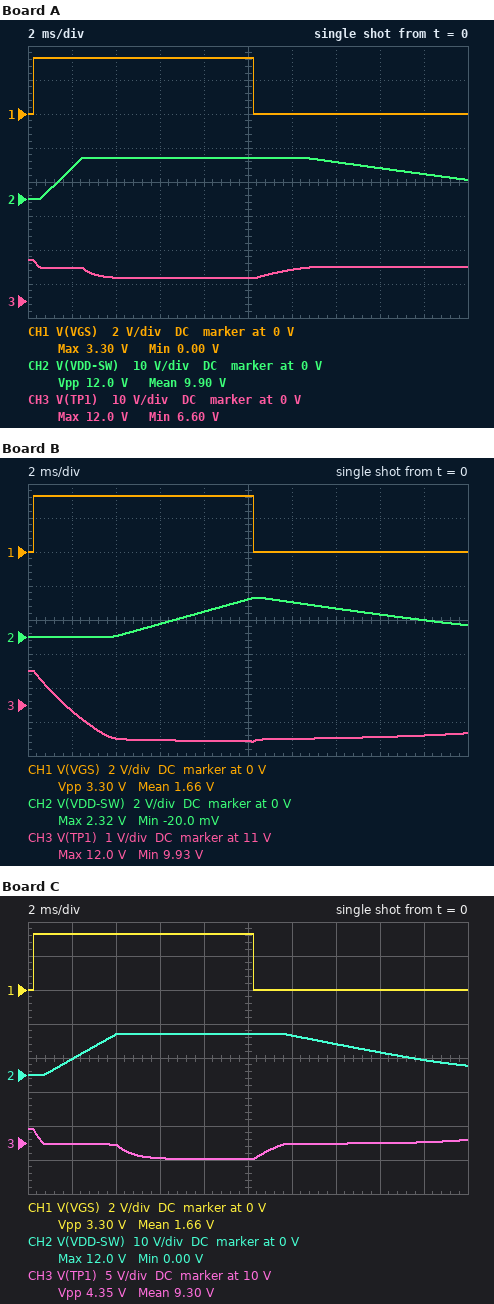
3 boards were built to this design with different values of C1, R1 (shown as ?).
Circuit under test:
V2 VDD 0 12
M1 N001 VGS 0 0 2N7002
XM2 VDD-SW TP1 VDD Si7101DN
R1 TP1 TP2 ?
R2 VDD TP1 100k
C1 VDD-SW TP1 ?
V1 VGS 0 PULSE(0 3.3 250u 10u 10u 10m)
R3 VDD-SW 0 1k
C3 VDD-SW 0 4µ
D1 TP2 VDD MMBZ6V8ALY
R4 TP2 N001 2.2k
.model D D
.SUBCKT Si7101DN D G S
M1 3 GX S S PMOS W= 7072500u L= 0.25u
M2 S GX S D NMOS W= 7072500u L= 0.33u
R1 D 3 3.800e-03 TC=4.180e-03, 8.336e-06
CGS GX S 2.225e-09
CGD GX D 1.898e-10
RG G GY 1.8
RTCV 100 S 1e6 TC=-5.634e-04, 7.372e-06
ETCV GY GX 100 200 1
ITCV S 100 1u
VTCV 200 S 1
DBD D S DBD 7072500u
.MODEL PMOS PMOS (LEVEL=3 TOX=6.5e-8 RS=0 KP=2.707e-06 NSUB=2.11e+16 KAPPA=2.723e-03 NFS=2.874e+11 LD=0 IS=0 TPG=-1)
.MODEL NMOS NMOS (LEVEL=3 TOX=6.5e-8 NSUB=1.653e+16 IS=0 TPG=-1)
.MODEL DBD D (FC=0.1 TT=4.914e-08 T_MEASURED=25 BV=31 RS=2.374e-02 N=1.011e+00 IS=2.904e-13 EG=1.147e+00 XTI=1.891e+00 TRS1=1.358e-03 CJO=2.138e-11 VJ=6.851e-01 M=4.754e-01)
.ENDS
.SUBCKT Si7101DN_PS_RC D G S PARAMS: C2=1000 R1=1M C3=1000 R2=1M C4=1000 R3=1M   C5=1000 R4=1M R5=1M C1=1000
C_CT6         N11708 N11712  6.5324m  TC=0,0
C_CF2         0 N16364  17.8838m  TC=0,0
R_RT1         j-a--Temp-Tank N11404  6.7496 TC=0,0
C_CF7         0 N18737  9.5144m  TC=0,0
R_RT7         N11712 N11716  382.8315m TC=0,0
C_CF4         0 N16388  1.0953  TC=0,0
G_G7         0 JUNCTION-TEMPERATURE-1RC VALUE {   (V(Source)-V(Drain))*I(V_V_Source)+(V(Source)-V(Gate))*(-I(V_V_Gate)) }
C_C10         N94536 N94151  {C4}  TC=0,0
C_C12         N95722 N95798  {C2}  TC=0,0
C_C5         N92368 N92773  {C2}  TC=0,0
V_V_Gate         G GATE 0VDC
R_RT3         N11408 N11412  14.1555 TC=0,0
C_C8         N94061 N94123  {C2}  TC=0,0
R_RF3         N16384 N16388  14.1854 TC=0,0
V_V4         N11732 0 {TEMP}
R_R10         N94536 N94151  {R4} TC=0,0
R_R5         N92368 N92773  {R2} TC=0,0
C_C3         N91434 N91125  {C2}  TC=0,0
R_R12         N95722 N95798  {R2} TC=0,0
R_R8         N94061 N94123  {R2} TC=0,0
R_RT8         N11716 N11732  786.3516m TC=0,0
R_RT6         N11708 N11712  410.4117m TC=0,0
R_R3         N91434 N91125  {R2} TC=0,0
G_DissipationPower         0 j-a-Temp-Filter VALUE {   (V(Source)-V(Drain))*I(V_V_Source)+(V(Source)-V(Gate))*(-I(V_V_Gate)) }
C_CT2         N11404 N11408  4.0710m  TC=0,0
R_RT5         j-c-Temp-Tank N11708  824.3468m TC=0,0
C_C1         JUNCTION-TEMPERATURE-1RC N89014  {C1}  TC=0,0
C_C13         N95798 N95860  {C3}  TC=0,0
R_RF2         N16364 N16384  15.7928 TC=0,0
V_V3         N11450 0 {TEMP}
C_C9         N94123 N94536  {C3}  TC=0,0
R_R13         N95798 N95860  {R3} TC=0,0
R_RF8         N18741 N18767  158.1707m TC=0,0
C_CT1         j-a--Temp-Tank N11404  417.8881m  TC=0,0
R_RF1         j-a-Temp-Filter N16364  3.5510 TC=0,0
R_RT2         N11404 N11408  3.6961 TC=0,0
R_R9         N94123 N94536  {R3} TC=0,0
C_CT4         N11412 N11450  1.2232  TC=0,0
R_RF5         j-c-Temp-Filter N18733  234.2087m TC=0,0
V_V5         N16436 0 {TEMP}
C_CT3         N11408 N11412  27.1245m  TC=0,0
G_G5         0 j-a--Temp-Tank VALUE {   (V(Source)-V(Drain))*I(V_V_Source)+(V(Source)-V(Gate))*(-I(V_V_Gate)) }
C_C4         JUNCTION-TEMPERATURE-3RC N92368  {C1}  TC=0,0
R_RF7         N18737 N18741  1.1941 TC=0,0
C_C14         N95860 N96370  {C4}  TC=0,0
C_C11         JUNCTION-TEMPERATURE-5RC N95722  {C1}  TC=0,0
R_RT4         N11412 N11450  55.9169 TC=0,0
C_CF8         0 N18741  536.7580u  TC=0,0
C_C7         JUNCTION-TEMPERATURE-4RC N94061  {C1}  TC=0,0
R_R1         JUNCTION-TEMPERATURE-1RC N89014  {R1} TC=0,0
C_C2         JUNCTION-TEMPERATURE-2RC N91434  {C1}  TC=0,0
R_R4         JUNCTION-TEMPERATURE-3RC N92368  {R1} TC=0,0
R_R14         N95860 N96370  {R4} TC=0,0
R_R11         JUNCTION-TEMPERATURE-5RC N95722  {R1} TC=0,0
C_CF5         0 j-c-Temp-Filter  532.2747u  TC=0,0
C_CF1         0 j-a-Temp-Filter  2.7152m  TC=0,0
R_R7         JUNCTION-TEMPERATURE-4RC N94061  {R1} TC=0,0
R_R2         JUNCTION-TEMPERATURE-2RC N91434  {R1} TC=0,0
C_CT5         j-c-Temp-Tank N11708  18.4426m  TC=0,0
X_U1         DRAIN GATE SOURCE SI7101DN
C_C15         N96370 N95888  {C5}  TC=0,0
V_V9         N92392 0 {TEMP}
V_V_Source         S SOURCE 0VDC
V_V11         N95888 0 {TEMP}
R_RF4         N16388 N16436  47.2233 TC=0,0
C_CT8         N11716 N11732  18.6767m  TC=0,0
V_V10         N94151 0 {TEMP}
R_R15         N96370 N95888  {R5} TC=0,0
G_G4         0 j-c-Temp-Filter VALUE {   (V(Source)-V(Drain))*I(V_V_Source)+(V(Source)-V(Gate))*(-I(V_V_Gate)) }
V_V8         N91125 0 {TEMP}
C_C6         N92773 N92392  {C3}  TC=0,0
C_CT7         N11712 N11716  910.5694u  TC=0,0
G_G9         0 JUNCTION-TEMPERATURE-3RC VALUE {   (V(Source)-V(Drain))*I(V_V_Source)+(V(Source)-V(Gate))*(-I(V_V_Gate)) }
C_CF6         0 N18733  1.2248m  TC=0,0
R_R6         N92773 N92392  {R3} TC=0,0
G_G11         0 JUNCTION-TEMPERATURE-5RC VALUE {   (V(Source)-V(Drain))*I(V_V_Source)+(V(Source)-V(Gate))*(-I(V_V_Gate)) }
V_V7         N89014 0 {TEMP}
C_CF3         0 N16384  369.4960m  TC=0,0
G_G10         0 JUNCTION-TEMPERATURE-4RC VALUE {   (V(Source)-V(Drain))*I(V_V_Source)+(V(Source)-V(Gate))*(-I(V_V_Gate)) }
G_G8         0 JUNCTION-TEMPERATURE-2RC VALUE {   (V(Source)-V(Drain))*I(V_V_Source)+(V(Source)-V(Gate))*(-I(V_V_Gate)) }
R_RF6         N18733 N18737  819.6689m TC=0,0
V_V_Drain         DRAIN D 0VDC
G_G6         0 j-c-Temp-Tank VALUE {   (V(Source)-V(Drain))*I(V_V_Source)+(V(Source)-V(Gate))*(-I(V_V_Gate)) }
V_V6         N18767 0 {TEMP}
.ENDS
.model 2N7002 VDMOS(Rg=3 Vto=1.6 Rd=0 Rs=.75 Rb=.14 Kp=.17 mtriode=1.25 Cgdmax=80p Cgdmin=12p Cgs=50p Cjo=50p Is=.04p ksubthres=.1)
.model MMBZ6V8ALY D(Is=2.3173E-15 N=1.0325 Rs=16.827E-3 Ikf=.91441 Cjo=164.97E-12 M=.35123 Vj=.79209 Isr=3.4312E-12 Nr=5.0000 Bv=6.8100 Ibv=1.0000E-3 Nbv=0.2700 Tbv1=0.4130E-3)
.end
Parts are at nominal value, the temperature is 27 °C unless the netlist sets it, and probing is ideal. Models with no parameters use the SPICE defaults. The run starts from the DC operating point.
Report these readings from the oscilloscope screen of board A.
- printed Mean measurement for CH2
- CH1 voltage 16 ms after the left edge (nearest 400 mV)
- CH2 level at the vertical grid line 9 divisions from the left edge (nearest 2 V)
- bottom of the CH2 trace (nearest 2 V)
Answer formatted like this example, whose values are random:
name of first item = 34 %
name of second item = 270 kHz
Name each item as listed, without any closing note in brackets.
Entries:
printed Mean measurement for CH2 = 9.90 V
CH1 voltage 16 ms after the left edge = 0 V
CH2 level at the vertical grid line 9 divisions from the left edge = 8 V
bottom of the CH2 trace = 0 V
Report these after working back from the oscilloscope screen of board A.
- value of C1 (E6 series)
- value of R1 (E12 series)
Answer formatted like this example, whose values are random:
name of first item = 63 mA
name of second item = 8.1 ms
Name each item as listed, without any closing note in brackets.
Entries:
value of C1 = 22 nF
value of R1 = 27 kΩ
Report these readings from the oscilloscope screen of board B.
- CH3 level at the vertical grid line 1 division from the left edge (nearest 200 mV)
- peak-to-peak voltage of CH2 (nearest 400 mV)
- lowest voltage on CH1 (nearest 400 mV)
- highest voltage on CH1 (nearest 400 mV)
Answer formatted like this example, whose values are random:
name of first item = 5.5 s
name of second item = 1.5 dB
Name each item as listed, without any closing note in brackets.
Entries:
CH3 level at the vertical grid line 1 division from the left edge = 10.8 V
peak-to-peak voltage of CH2 = 2.4 V
lowest voltage on CH1 = 0 V
highest voltage on CH1 = 3.2 V
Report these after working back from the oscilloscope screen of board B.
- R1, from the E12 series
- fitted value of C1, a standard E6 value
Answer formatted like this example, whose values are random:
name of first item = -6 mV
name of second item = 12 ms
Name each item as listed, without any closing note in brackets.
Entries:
R1, from the E12 series = 82 kΩ
fitted value of C1, a standard E6 value = 100 nF
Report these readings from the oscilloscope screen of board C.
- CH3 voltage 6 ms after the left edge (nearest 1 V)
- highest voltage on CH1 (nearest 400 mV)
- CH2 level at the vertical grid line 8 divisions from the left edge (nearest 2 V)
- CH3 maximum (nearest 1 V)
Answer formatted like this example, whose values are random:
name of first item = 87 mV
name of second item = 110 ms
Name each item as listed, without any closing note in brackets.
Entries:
CH3 voltage 6 ms after the left edge = 8 V
highest voltage on CH1 = 3.2 V
CH2 level at the vertical grid line 8 divisions from the left edge = 6 V
CH3 maximum = 12 V
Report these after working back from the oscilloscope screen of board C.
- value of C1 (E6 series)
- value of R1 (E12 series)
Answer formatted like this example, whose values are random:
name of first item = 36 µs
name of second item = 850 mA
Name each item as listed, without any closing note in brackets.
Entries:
value of C1 = 15 nF
value of R1 = 56 kΩ
